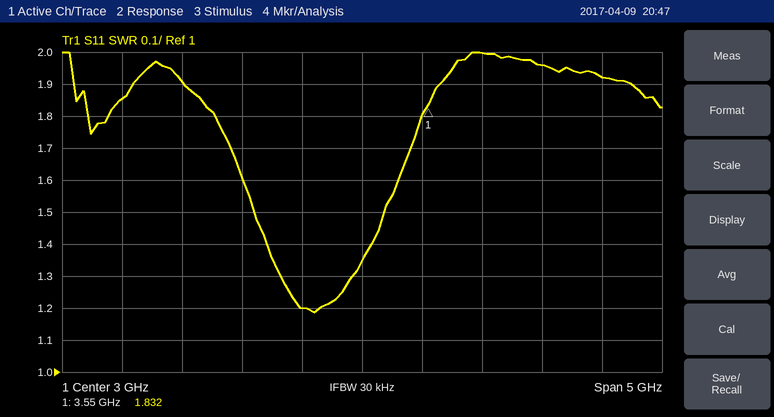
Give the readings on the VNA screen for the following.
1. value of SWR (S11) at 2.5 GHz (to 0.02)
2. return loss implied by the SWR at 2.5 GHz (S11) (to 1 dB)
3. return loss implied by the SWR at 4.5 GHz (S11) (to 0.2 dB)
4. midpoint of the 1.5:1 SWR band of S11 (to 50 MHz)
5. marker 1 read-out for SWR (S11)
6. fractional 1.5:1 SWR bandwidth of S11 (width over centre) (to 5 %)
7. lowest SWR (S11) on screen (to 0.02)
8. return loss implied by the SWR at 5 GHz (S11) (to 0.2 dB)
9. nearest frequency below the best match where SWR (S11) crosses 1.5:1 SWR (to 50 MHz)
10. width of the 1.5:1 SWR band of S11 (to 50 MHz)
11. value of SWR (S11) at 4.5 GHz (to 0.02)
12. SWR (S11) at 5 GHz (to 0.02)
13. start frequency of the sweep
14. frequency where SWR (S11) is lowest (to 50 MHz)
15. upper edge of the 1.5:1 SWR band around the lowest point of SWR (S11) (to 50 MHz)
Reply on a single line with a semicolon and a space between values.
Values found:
1.20; 21 dB; 9.8 dB; 2.65 GHz; 1.832; 40 %; 1.18; 10.0 dB; 2.10 GHz; 1.10 GHz; 1.96; 1.92; 500 MHz; 2.60 GHz; 3.20 GHz
